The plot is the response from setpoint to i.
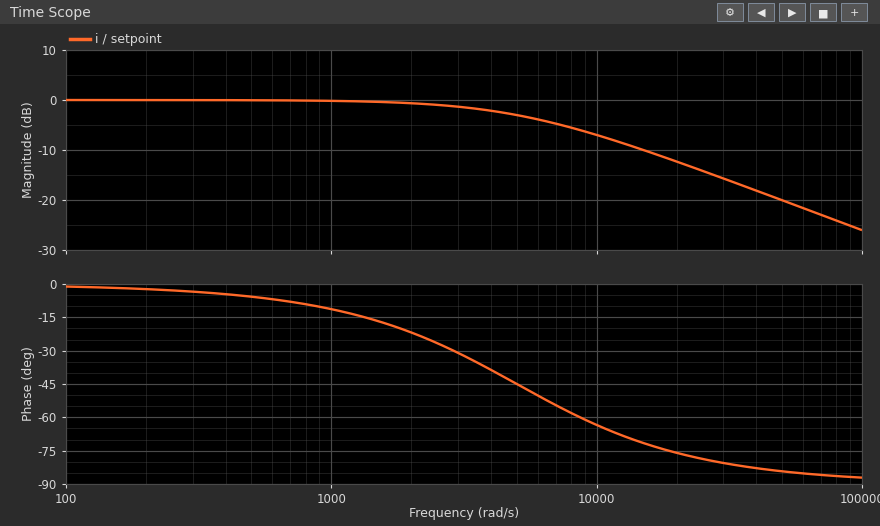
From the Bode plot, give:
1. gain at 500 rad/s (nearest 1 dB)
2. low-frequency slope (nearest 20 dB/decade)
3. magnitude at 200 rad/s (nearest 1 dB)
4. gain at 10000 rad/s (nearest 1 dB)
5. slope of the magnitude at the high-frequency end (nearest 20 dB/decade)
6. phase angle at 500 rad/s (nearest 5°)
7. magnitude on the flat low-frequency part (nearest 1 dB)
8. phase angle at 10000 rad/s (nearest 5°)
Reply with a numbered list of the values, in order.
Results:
1. 0 dB
2. 0 dB/decade
3. 0 dB
4. -7 dB
5. -20 dB/decade
6. -5°
7. 0 dB
8. -65°
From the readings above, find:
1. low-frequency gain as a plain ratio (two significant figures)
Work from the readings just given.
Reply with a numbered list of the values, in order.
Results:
1. 1.0
